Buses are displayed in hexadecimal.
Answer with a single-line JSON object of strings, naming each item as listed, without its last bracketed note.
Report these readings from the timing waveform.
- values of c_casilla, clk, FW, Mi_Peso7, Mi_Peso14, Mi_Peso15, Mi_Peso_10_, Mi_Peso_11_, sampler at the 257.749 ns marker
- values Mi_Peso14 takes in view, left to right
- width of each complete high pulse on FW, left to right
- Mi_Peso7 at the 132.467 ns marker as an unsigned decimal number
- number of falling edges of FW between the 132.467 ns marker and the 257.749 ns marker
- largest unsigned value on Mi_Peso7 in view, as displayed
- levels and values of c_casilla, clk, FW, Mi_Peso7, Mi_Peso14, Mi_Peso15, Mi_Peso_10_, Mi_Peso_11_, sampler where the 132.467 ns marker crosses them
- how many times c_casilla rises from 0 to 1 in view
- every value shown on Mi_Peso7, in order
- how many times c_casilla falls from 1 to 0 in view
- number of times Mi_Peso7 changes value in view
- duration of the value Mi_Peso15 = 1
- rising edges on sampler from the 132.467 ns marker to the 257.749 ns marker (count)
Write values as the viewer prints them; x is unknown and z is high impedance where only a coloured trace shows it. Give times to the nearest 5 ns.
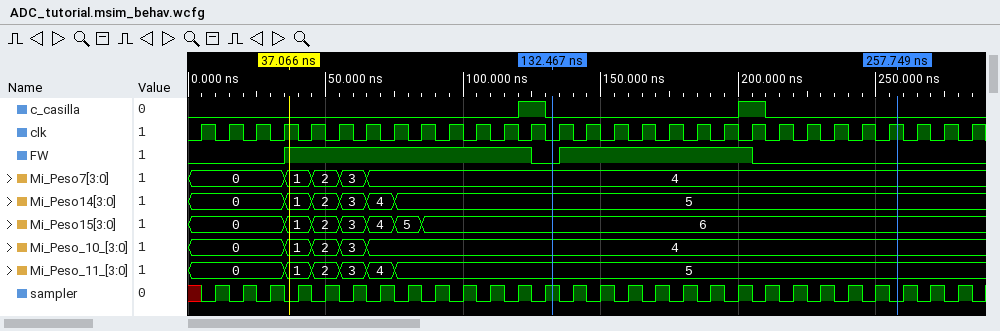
{"values of c_casilla, clk, FW, Mi_Peso7, Mi_Peso14, Mi_Peso15, Mi_Peso_10_, Mi_Peso_11_, sampler at the 257.749 ns marker": "c_casilla=0, clk=1, FW=0, Mi_Peso7=4, Mi_Peso14=5, Mi_Peso15=6, Mi_Peso_10_=4, Mi_Peso_11_=5, sampler=0", "values Mi_Peso14 takes in view, left to right": "0, 1, 2, 3, 4, 5", "width of each complete high pulse on FW, left to right": "90 ns, 70 ns", "Mi_Peso7 at the 132.467 ns marker as an unsigned decimal number": "4", "number of falling edges of FW between the 132.467 ns marker and the 257.749 ns marker": "1", "largest unsigned value on Mi_Peso7 in view, as displayed": "4", "levels and values of c_casilla, clk, FW, Mi_Peso7, Mi_Peso14, Mi_Peso15, Mi_Peso_10_, Mi_Peso_11_, sampler where the 132.467 ns marker crosses them": "c_casilla=0, clk=0, FW=0, Mi_Peso7=4, Mi_Peso14=5, Mi_Peso15=6, Mi_Peso_10_=4, Mi_Peso_11_=5, sampler=1", "how many times c_casilla rises from 0 to 1 in view": "2", "every value shown on Mi_Peso7, in order": "0, 1, 2, 3, 4", "how many times c_casilla falls from 1 to 0 in view": "2", "number of times Mi_Peso7 changes value in view": "4", "duration of the value Mi_Peso15 = 1": "10 ns", "rising edges on sampler from the 132.467 ns marker to the 257.749 ns marker": "12"}
